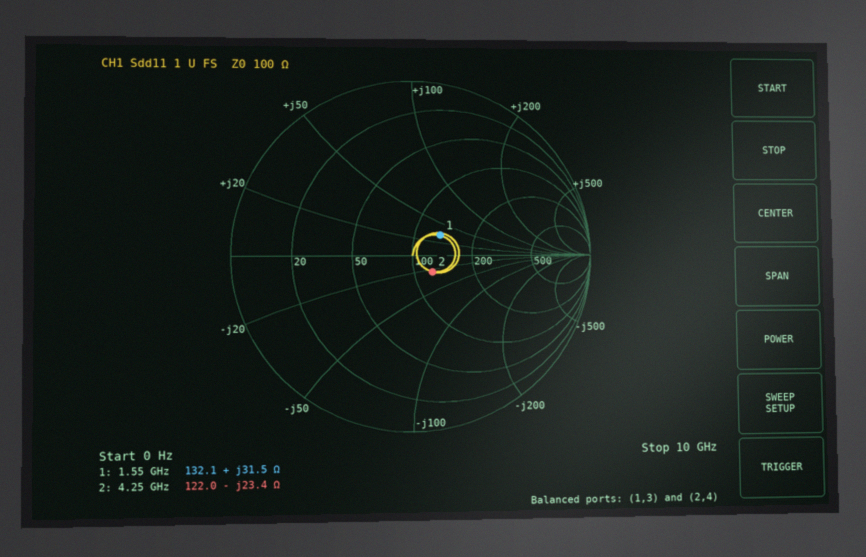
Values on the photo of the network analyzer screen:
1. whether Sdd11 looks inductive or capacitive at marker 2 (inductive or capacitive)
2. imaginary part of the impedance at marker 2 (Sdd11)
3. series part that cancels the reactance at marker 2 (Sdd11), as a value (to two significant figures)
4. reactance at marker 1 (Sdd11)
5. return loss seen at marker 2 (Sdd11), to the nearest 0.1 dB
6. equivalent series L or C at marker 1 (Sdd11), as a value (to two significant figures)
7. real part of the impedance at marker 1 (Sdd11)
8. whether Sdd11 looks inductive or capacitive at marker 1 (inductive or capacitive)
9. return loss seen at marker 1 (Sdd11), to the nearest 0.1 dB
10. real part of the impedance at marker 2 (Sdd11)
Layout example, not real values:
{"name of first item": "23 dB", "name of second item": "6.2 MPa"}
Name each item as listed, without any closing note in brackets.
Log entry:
{"whether Sdd11 looks inductive or capacitive at marker 2": "capacitive", "imaginary part of the impedance at marker 2": "-23.4 Ω", "series part that cancels the reactance at marker 2 (Sdd11), as a value": "880 pH", "reactance at marker 1": "+31.5 Ω", "return loss seen at marker 2 (Sdd11), to the nearest 0.1 dB": "16.8 dB", "equivalent series L or C at marker 1 (Sdd11), as a value": "3.2 nH", "real part of the impedance at marker 1": "132.1 Ω", "whether Sdd11 looks inductive or capacitive at marker 1": "inductive", "return loss seen at marker 1 (Sdd11), to the nearest 0.1 dB": "14.3 dB", "real part of the impedance at marker 2": "122.0 Ω"}
